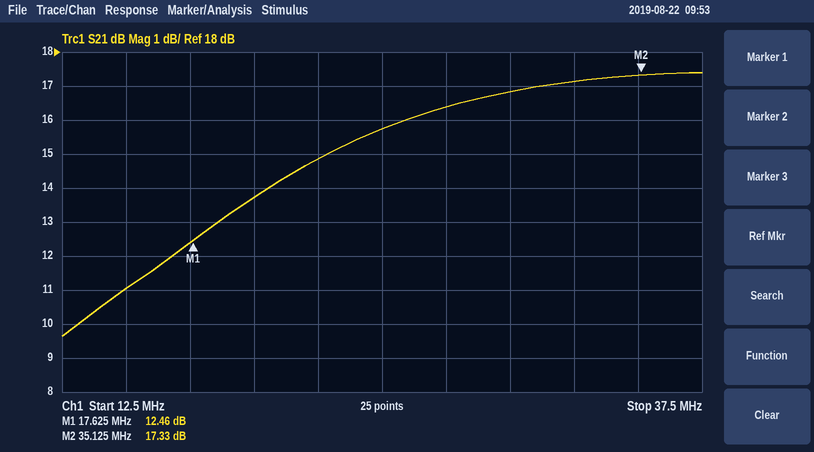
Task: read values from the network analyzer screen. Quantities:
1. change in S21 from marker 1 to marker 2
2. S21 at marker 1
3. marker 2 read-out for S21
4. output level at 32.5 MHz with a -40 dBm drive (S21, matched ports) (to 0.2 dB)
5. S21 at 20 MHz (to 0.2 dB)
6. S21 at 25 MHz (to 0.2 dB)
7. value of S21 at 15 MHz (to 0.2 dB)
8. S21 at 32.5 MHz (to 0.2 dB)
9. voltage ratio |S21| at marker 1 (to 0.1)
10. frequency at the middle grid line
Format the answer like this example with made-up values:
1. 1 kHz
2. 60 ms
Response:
1. 4.87 dB
2. 12.46 dB
3. 17.33 dB
4. -22.8 dBm
5. 13.8 dB
6. 15.8 dB
7. 11.0 dB
8. 17.2 dB
9. 4.2
10. 25 MHz
